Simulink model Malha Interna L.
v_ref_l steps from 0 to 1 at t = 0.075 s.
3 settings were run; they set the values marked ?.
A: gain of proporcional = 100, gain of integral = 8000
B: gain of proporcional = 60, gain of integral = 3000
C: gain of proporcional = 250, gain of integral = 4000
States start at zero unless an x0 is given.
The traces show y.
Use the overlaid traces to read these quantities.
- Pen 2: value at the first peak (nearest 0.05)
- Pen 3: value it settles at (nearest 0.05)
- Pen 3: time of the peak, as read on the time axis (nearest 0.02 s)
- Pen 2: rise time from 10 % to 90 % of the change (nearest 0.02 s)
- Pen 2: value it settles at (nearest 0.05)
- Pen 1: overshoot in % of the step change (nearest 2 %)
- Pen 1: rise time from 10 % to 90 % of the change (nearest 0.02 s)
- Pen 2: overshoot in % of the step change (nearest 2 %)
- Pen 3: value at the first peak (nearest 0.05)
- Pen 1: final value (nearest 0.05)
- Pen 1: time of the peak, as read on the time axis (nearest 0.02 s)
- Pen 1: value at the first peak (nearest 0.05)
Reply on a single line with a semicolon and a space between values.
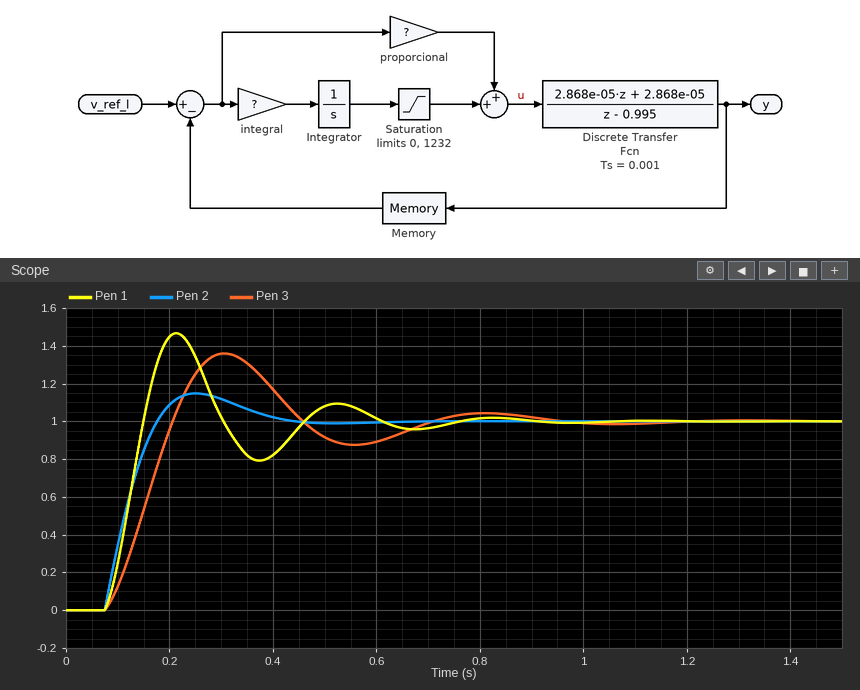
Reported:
1.15; 1.00; 0.30 s; 0.08 s; 1.00; 46 %; 0.06 s; 14 %; 1.35; 1.00; 0.22 s; 1.45
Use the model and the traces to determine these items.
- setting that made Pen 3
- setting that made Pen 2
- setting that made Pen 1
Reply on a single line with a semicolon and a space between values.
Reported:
B; C; A
